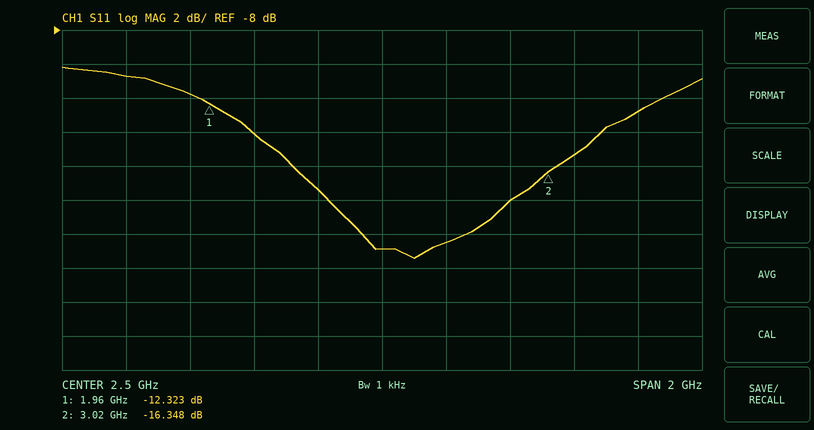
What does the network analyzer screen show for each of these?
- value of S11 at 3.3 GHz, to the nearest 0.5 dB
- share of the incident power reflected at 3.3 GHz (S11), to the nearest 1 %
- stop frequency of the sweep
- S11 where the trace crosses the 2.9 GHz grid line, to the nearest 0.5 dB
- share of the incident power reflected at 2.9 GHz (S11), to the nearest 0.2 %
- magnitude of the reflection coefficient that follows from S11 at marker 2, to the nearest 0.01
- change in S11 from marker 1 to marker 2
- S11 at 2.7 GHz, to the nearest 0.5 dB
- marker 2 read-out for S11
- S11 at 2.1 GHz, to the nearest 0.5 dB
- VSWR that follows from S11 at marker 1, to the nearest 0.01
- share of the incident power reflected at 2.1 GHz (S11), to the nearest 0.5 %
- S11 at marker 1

-13.0 dB
5 %
3.5 GHz
-18.0 dB
1.6 %
0.15
-4.025 dB
-20.5 dB
-16.348 dB
-14.0 dB
1.64
4.0 %
-12.323 dB
